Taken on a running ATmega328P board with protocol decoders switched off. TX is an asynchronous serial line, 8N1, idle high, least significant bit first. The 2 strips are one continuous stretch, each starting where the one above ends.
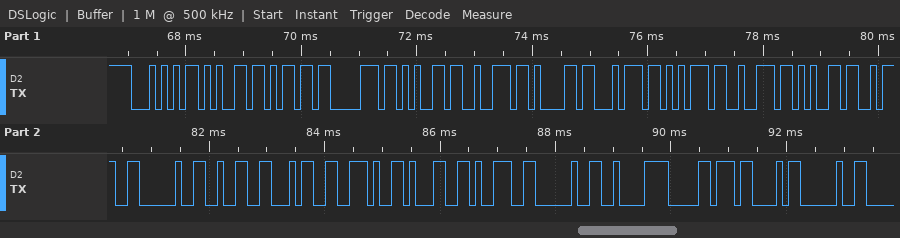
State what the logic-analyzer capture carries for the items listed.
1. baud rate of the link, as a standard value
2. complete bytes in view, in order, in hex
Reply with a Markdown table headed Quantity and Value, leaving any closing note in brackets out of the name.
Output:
| Quantity | Value |
|---|---|
| baud rate of the link, as a standard value | 9600 baud |
| complete bytes in view, in order, in hex | 0x54 0x65 0x6D 0x70 0x65 0x72 0x61 0x74 0x75 0x72 0x65 0x3A 0x20 0x32 0x34 0x2E 0x31 0x39 0x20 0xC2 0xB0 0x43 0x20 |
